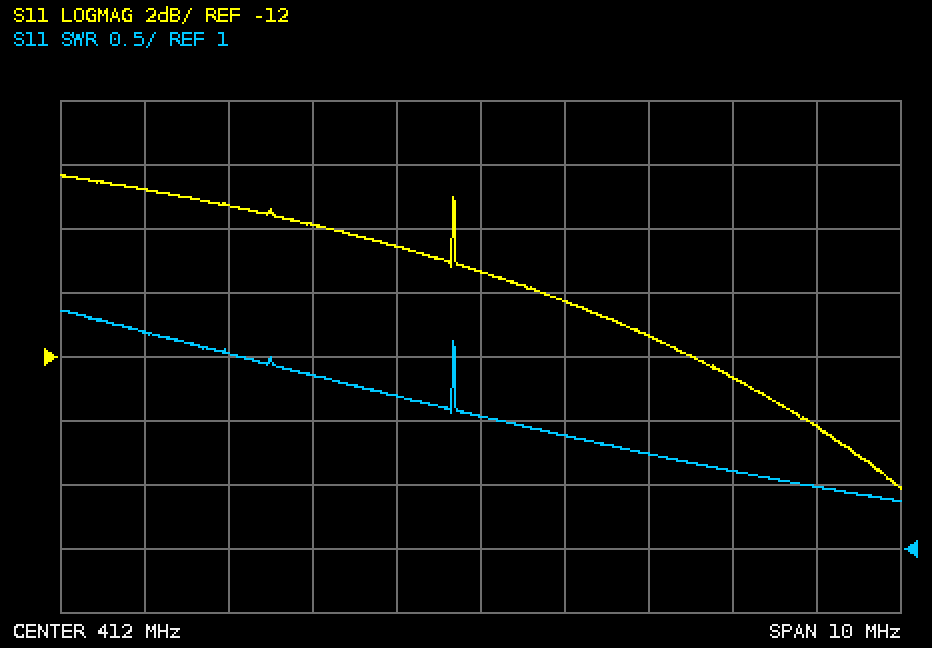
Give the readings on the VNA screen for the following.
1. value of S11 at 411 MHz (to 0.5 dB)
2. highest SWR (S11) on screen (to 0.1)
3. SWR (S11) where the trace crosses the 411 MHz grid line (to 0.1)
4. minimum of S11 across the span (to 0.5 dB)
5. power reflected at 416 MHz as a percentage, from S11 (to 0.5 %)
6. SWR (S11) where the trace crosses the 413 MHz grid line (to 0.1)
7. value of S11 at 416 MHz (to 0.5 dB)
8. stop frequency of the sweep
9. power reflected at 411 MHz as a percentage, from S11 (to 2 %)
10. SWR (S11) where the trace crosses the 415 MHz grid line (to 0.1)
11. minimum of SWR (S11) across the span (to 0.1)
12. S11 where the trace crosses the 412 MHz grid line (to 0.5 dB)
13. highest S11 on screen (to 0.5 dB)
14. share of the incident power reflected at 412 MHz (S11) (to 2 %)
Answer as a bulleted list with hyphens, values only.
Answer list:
- -8.5 dB
- 2.9
- 2.2
- -16.0 dB
- 4.0 %
- 1.9
- -14.0 dB
- 417 MHz
- 14 %
- 1.6
- 1.4
- -9.5 dB
- -6.5 dB
- 12 %
